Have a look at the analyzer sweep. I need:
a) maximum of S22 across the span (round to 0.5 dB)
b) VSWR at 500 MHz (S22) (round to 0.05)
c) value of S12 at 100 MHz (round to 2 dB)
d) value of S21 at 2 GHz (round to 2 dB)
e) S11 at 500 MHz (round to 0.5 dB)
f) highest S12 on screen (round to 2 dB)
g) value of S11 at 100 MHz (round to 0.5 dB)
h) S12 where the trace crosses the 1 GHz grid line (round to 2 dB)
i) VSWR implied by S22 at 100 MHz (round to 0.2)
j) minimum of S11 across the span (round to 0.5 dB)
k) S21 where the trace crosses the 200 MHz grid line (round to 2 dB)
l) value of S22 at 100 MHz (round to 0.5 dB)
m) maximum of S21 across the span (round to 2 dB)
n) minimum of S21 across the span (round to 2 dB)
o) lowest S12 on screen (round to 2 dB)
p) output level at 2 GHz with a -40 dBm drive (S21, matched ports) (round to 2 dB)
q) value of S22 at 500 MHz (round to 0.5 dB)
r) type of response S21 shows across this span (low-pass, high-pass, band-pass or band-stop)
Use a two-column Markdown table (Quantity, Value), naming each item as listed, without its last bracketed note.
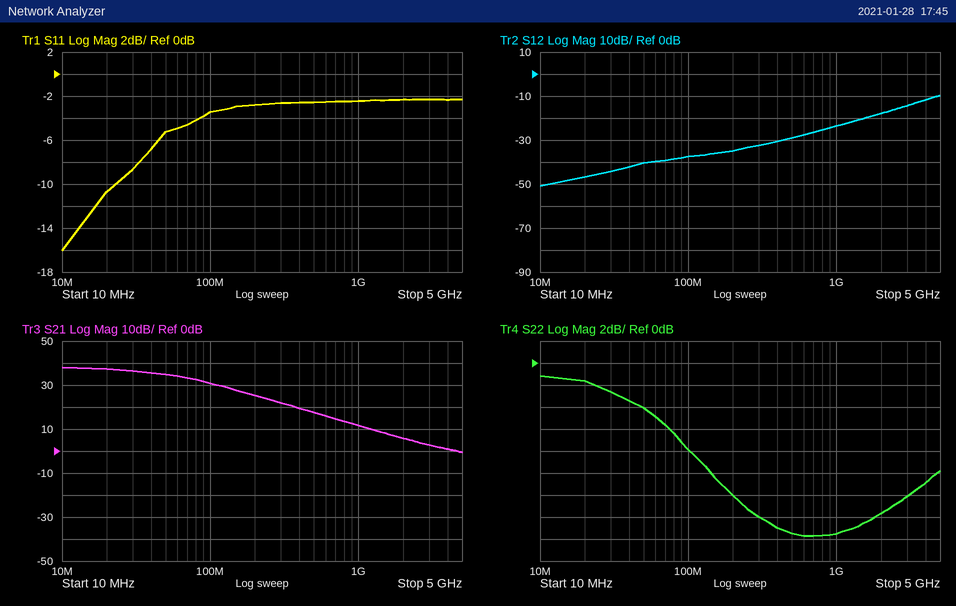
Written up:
| Quantity | Value |
|---|---|
| maximum of S22 across the span | -1.0 dB |
| VSWR at 500 MHz (S22) | 1.40 |
| value of S12 at 100 MHz | -38 dB |
| value of S21 at 2 GHz | 6 dB |
| S11 at 500 MHz | -2.5 dB |
| highest S12 on screen | -10 dB |
| value of S11 at 100 MHz | -3.5 dB |
| S12 where the trace crosses the 1 GHz grid line | -24 dB |
| VSWR implied by S22 at 100 MHz | 2.4 |
| minimum of S11 across the span | -16.0 dB |
| S21 where the trace crosses the 200 MHz grid line | 26 dB |
| value of S22 at 100 MHz | -8.0 dB |
| maximum of S21 across the span | 38 dB |
| minimum of S21 across the span | 0 dB |
| lowest S12 on screen | -50 dB |
| output level at 2 GHz with a -40 dBm drive (S21, matched ports) | -34 dBm |
| value of S22 at 500 MHz | -15.5 dB |
| type of response S21 shows across this span | low-pass |
